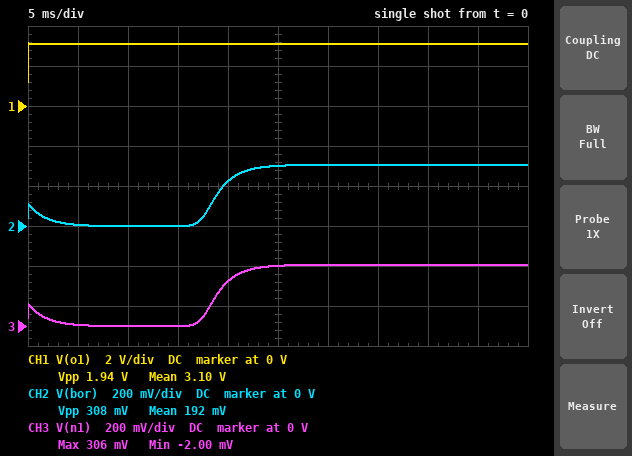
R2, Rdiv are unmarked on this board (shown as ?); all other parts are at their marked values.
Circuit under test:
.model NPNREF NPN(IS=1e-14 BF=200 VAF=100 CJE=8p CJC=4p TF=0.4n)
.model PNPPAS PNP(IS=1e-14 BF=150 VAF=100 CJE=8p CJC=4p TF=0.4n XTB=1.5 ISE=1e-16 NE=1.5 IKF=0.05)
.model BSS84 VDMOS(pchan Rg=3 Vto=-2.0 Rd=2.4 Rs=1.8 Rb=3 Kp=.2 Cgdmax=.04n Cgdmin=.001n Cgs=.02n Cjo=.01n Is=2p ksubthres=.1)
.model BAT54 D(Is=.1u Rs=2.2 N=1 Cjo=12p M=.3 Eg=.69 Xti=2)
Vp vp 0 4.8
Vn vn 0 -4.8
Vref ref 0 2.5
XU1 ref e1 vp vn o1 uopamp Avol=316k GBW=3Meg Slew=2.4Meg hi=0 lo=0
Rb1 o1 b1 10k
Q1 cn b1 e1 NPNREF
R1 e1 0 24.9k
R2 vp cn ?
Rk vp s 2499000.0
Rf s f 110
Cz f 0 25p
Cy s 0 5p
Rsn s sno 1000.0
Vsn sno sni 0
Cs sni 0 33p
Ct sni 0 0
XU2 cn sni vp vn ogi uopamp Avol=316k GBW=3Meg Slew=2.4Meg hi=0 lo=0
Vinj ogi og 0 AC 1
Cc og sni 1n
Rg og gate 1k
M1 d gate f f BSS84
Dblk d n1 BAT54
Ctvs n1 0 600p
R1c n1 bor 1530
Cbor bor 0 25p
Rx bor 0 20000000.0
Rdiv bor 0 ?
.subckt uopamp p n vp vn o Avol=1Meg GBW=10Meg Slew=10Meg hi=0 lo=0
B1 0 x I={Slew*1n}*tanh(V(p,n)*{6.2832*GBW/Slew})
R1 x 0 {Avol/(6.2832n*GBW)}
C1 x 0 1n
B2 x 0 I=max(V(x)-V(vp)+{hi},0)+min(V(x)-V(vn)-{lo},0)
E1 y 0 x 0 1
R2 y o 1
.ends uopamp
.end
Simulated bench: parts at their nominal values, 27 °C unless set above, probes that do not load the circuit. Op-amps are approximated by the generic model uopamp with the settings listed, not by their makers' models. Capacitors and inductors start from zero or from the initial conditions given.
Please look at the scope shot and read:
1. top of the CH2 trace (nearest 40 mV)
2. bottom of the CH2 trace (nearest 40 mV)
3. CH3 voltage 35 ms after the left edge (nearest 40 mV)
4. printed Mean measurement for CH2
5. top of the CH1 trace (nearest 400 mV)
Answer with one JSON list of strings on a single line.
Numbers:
["320 mV", "0 V", "320 mV", "192 mV", "3.2 V"]
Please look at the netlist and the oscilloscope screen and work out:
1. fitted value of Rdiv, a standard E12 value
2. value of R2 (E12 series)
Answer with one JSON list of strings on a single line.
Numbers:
["3.3 MΩ", "2.7 kΩ"]
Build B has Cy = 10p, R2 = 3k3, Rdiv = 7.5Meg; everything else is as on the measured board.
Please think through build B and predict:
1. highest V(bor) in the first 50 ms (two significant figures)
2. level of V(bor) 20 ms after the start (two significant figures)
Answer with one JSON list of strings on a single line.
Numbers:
["720 mV", "570 mV"]
